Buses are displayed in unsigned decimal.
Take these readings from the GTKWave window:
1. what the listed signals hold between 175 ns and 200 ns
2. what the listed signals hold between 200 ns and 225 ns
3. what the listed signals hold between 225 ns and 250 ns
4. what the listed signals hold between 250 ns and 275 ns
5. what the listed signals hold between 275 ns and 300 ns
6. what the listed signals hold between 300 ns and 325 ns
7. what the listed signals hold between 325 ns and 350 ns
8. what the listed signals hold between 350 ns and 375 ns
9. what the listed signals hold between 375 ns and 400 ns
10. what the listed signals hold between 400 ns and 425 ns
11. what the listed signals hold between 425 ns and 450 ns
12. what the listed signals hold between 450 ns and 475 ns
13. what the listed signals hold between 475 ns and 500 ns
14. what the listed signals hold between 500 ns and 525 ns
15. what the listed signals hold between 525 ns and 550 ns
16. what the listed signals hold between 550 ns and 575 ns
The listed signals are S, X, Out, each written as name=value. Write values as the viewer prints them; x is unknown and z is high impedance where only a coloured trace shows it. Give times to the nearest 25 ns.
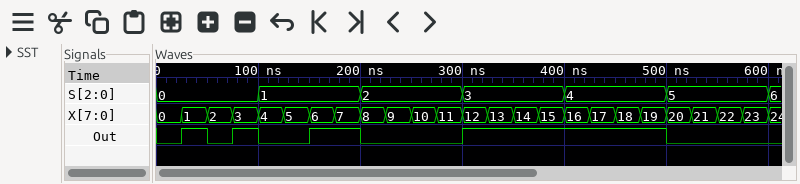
S=1, X=7, Out=1
S=2, X=8, Out=0
S=2, X=9, Out=0
S=2, X=10, Out=0
S=2, X=11, Out=0
S=3, X=12, Out=1
S=3, X=13, Out=1
S=3, X=14, Out=1
S=3, X=15, Out=1
S=4, X=16, Out=1
S=4, X=17, Out=1
S=4, X=18, Out=1
S=4, X=19, Out=1
S=5, X=20, Out=0
S=5, X=21, Out=0
S=5, X=22, Out=0
